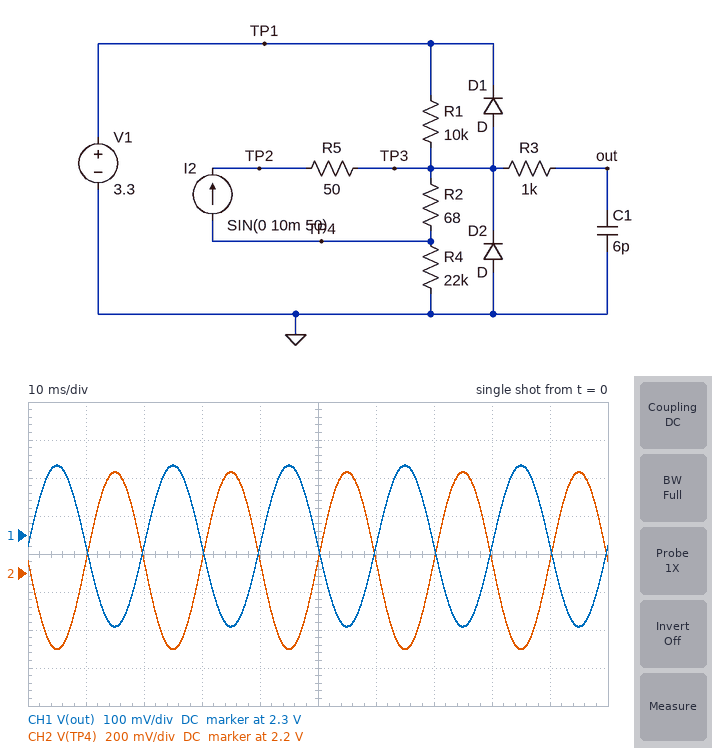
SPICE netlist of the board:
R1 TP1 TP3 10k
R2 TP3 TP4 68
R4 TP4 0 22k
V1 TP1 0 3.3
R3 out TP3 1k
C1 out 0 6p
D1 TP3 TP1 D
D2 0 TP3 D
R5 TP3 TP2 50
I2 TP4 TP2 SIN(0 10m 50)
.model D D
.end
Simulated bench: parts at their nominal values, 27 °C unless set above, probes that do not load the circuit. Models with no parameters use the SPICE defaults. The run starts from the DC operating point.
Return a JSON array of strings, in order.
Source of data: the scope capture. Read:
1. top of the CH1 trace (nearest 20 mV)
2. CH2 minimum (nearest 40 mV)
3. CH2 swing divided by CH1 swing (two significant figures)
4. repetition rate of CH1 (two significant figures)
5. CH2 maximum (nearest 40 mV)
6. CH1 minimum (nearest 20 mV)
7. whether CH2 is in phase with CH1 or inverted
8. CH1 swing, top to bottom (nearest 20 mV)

["2.48 V", "1.80 V", "2.2", "50 Hz", "2.72 V", "2.06 V", "inverted", "420 mV"]
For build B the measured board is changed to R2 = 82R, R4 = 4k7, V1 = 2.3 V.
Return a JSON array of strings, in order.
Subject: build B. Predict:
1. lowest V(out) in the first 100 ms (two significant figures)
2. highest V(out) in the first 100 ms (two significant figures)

["190 mV", "1.3 V"]
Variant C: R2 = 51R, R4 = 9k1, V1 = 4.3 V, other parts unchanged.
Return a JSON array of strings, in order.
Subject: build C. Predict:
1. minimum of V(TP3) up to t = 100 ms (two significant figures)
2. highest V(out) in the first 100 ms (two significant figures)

["1.8 V", "2.3 V"]
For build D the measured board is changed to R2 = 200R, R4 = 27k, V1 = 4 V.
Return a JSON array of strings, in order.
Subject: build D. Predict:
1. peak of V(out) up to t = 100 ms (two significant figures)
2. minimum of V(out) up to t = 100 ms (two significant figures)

["3.5 V", "2.4 V"]
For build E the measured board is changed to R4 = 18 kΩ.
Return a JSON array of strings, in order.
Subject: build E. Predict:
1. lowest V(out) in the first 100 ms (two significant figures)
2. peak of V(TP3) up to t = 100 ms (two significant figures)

["1.9 V", "2.4 V"]
